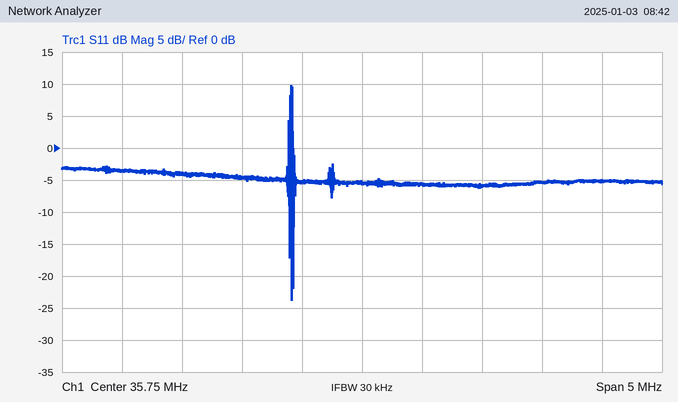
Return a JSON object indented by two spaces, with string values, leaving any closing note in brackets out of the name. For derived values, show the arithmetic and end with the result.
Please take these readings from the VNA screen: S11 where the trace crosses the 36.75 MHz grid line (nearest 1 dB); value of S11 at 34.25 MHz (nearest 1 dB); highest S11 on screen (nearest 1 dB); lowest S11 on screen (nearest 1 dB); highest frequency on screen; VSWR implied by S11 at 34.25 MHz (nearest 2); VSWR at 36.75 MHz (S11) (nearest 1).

{
  "S11 where the trace crosses the 36.75 MHz grid line": "-6 dB",
  "value of S11 at 34.25 MHz": "-4 dB",
  "highest S11 on screen": "10 dB",
  "lowest S11 on screen": "-24 dB",
  "highest frequency on screen": "38.25 MHz",
  "VSWR implied by S11 at 34.25 MHz": "|Γ| = 10^(-4/20) = 0.6310; VSWR = (1 + 0.6310)/(1 − 0.6310) ≈ 4",
  "VSWR at 36.75 MHz (S11)": "|Γ| = 10^(-6/20) = 0.5012; VSWR = (1 + 0.5012)/(1 − 0.5012) ≈ 3"
}
